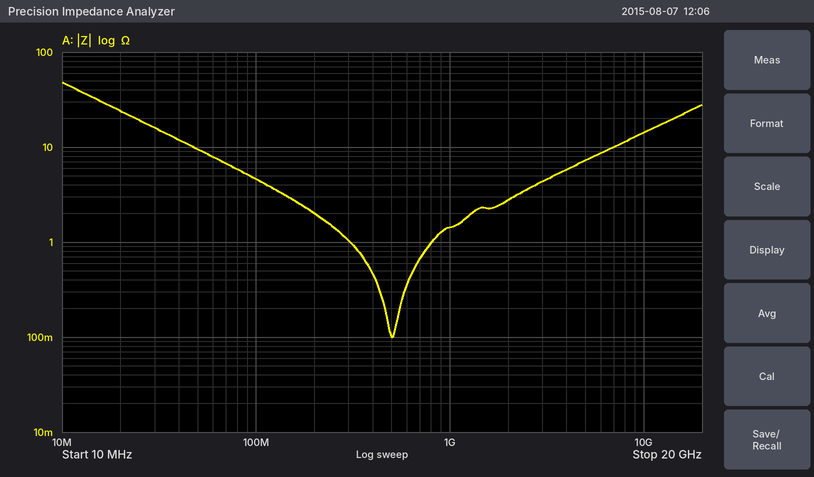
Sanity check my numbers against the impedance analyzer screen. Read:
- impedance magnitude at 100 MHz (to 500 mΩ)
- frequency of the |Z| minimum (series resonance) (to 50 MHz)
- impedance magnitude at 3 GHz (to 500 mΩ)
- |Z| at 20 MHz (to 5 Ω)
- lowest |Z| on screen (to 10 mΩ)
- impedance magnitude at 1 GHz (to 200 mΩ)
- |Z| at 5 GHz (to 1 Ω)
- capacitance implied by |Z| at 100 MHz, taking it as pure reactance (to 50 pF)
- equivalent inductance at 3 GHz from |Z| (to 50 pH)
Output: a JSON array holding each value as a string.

["4.5 Ω", "500 MHz", "4.5 Ω", "25 Ω", "100 mΩ", "1.4 Ω", "7 Ω", "350 pF", "250 pH"]
